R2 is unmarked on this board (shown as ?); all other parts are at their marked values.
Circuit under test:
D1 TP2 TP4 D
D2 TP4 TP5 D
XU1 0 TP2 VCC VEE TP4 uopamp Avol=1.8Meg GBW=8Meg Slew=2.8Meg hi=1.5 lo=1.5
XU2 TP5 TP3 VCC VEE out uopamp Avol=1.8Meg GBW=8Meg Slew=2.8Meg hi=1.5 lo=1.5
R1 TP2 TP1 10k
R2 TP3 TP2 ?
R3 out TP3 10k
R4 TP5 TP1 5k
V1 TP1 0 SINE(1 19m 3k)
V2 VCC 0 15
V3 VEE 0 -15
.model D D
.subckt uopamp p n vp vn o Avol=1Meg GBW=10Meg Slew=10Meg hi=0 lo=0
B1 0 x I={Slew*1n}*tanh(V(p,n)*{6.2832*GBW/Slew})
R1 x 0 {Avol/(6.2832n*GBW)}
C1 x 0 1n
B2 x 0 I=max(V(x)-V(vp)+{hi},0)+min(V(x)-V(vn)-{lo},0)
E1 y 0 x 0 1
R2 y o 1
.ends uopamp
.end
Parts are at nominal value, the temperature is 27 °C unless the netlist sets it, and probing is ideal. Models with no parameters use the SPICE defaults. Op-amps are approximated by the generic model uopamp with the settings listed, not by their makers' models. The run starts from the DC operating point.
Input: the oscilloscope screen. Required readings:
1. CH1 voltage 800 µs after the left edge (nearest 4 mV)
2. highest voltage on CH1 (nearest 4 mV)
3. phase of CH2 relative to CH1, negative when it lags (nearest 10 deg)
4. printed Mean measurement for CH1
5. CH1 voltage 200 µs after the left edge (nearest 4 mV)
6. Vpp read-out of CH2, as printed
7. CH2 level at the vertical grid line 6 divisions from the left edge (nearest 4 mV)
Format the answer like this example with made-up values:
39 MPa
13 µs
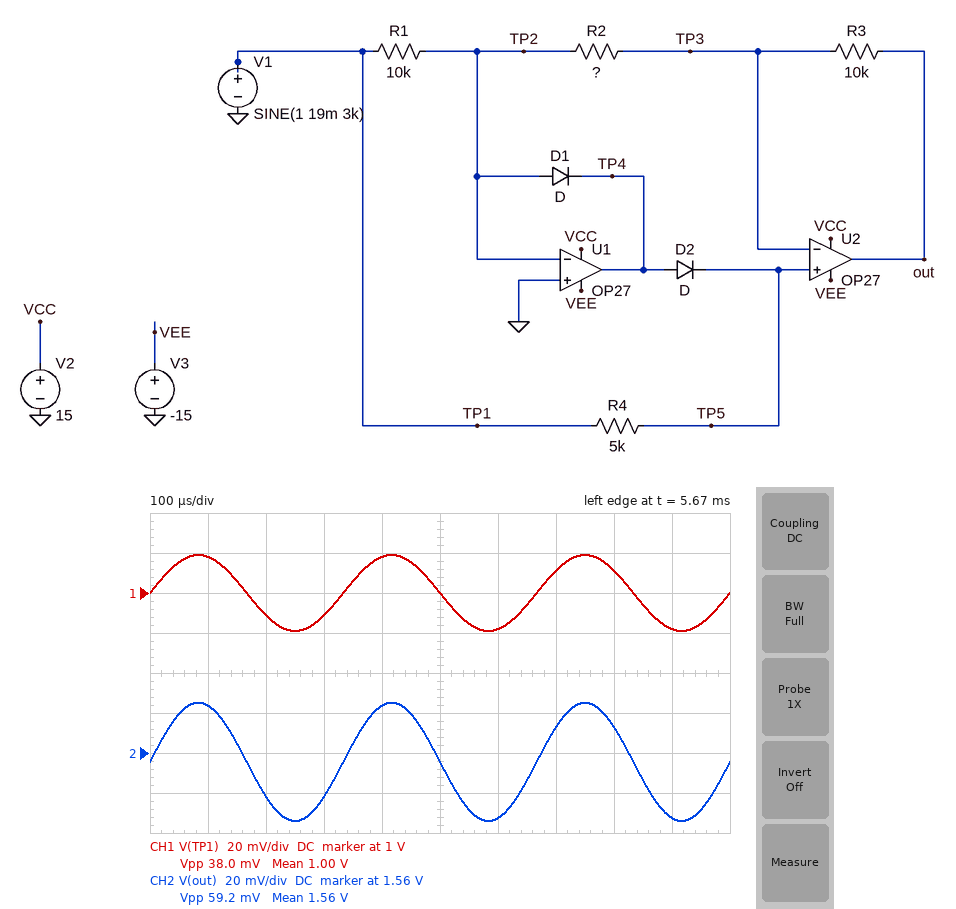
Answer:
1.012 V
1.020 V
0 deg
1.00 V
988 mV
59.2 mV
1.528 V
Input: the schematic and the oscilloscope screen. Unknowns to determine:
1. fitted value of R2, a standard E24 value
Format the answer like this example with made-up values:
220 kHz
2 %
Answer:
18 kΩ
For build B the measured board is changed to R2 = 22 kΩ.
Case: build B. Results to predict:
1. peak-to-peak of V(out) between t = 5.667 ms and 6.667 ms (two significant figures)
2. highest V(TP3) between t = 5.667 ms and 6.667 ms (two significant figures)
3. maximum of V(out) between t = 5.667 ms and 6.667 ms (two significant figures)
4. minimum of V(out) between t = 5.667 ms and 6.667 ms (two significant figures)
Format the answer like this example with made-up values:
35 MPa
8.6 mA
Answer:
55 mV
1.0 V
1.5 V
1.4 V
